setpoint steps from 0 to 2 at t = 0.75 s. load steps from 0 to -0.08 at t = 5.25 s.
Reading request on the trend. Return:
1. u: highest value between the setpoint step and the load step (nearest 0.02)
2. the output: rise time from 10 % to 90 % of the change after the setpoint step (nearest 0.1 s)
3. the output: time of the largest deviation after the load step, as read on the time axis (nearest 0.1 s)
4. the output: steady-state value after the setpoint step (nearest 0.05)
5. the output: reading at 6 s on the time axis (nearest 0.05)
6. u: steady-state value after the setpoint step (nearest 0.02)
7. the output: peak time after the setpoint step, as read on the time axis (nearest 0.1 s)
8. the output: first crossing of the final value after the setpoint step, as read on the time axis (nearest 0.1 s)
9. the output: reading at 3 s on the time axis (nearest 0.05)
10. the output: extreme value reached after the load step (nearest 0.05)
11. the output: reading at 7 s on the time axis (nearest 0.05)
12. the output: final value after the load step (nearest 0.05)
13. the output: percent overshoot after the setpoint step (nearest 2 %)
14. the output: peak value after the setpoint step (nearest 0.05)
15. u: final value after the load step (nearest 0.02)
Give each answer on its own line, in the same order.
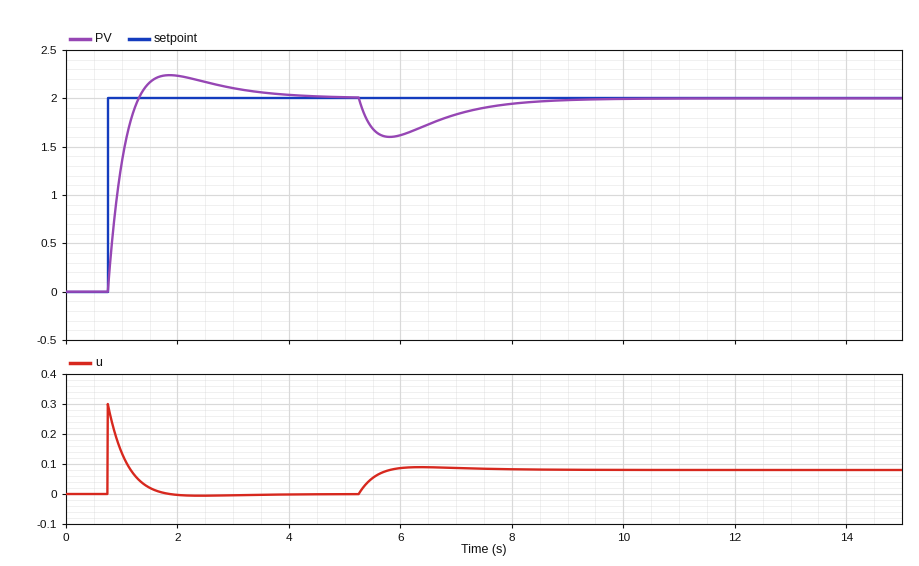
0.30
0.4 s
5.8 s
2.00
1.60
0.00
1.9 s
1.3 s
2.10
1.60
1.85
2.00
12 %
2.25
0.08
